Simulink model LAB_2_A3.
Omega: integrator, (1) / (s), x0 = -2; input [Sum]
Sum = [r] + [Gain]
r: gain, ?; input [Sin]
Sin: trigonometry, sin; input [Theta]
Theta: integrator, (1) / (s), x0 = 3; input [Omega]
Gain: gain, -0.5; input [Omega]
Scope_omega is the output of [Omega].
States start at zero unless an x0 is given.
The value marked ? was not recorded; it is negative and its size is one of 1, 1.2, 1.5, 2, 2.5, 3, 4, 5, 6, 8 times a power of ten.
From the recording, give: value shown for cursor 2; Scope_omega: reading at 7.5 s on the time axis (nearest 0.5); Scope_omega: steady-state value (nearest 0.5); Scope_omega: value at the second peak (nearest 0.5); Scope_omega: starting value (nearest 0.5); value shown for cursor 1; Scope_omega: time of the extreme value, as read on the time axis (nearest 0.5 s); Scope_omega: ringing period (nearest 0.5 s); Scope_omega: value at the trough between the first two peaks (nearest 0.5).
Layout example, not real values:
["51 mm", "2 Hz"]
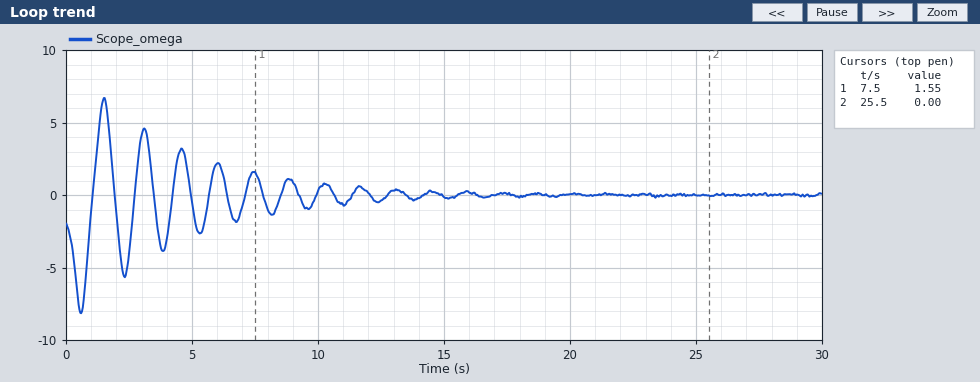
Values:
["0.00", "1.5", "0.0", "4.5", "-2.0", "1.55", "1.5 s", "1.5 s", "-5.5"]
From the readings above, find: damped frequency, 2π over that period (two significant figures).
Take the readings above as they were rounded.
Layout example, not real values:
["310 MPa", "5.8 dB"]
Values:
["4.2 rad/s"]
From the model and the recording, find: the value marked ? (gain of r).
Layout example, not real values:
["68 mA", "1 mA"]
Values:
["-20"]
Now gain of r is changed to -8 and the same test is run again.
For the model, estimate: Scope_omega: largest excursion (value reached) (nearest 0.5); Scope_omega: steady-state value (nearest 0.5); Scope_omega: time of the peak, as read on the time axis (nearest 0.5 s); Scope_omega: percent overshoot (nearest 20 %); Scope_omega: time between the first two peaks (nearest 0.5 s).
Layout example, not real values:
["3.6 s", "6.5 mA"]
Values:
["3.5", "0.0", "2.0 s", "180 %", "2.5 s"]
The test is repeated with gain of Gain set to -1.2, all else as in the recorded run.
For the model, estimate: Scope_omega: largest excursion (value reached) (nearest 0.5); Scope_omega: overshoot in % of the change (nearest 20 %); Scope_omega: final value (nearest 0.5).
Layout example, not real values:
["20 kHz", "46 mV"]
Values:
["4.5", "220 %", "0.0"]
